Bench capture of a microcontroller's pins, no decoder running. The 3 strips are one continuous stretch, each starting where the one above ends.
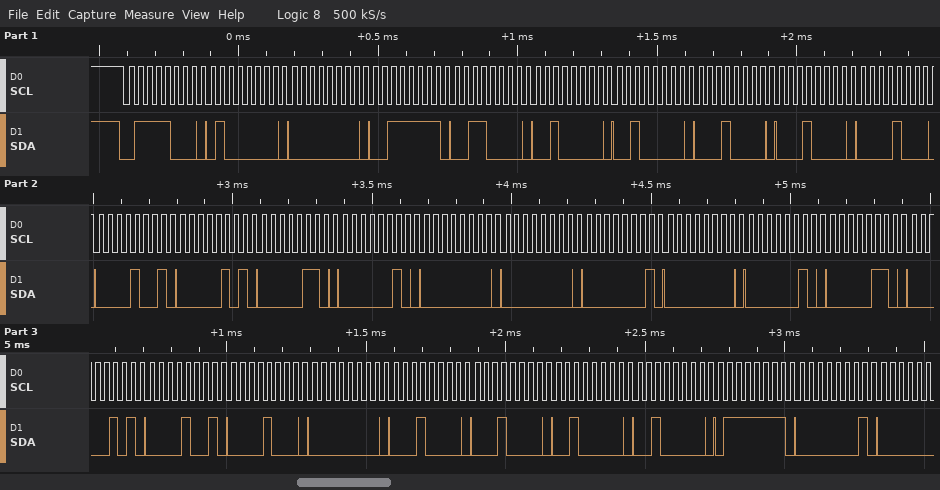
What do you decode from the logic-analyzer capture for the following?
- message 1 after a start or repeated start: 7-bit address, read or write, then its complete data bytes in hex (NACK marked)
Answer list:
0x3C write: 40 00 3F 30 20 20 10 10 08 09 05 06 02 00 00 01 00 02 06 05 09 08 00 10 10 20 20 7F 01
